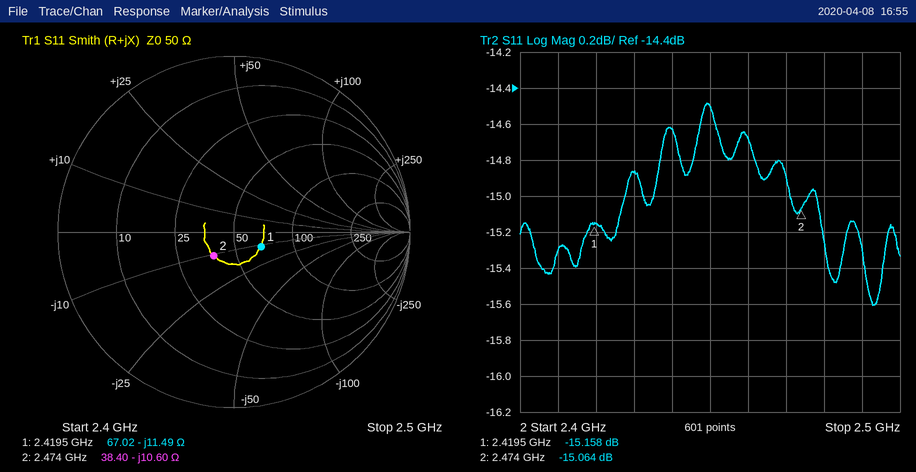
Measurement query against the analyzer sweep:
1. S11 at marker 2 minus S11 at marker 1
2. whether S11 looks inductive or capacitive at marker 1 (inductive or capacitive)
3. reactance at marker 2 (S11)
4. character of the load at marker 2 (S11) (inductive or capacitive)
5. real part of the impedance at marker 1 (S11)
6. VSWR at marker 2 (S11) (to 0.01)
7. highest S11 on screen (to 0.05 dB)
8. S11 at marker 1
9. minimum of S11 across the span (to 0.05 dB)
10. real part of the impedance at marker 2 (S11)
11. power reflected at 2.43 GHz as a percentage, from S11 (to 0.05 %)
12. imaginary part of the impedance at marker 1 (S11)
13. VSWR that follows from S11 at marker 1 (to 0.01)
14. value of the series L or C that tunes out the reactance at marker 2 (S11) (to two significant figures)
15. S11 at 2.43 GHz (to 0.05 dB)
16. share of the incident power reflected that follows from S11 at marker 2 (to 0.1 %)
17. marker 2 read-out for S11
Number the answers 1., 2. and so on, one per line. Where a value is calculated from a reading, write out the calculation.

1. -15.064 − (-15.158) = 0.094 dB
2. capacitive
3. -10.60 Ω
4. capacitive
5. 67.02 Ω
6. 1.43
7. -14.50 dB
8. -15.158 dB
9. -15.60 dB
10. 38.40 Ω
11. 10^(-14.85/10) ≈ 3.27 %, so 3.25 % to the nearest 0.05 %
12. -11.49 Ω
13. (1 + 0.1746)/(1 − 0.1746) ≈ 1.42
14. L = 10.6 Ω/(2π × 2.474 GHz) ≈ 682 pH, so 680 pH to two significant figures
15. -14.85 dB
16. 10^(-15.064/10) ≈ 3.1 %
17. -15.064 dB
